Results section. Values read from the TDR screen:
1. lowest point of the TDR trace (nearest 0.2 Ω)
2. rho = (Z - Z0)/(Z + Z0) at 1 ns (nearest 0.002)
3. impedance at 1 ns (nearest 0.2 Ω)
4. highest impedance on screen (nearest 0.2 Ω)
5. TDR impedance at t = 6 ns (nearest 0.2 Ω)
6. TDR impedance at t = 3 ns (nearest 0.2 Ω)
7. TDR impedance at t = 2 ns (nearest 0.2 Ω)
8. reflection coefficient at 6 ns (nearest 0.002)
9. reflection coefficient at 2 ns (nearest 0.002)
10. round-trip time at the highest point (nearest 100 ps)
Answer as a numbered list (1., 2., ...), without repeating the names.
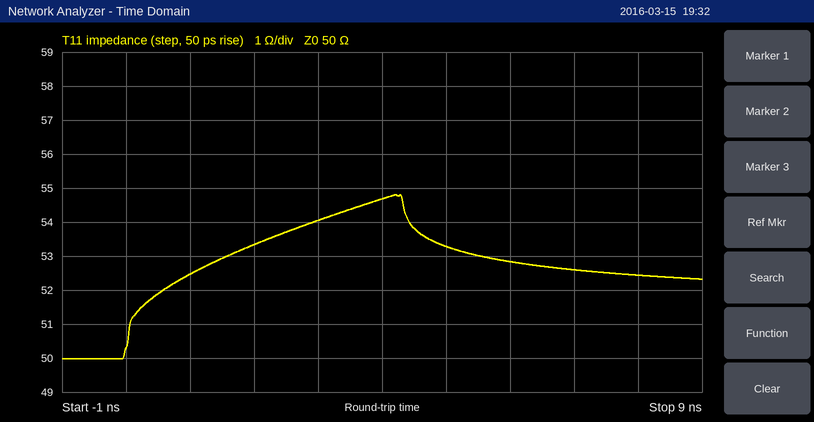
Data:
1. 50.0 Ω
2. +0.024
3. 52.4 Ω
4. 54.8 Ω
5. 52.8 Ω
6. 54.0 Ω
7. 53.4 Ω
8. +0.028
9. +0.032
10. 4.2 ns
